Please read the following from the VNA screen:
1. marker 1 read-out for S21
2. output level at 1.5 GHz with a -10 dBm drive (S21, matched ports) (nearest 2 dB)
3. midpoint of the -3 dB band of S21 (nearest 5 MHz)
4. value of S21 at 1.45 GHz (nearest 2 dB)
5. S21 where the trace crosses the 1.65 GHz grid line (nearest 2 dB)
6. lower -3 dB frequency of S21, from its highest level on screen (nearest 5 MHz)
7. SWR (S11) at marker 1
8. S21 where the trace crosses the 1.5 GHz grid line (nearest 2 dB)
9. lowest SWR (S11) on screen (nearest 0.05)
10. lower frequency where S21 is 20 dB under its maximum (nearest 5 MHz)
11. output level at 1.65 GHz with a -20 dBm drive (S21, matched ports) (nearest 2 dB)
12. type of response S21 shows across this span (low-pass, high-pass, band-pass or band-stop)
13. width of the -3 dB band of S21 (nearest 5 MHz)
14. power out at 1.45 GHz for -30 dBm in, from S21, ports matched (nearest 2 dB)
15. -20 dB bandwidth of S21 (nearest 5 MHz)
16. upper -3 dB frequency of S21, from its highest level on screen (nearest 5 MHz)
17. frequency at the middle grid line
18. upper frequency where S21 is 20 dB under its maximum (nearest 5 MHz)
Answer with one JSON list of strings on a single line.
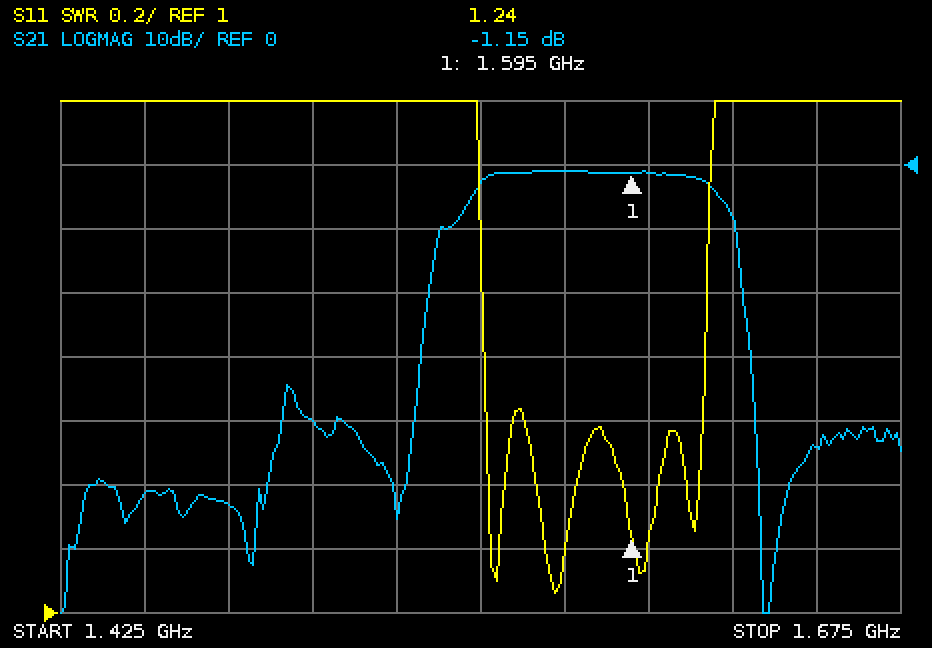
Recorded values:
["-1.15 dB", "-50 dBm", "1.585 GHz", "-52 dB", "-44 dB", "1.550 GHz", "1.24", "-40 dB", "1.05", "1.535 GHz", "-64 dBm", "band-pass", "70 MHz", "-82 dBm", "95 MHz", "1.620 GHz", "1.55 GHz", "1.630 GHz"]
